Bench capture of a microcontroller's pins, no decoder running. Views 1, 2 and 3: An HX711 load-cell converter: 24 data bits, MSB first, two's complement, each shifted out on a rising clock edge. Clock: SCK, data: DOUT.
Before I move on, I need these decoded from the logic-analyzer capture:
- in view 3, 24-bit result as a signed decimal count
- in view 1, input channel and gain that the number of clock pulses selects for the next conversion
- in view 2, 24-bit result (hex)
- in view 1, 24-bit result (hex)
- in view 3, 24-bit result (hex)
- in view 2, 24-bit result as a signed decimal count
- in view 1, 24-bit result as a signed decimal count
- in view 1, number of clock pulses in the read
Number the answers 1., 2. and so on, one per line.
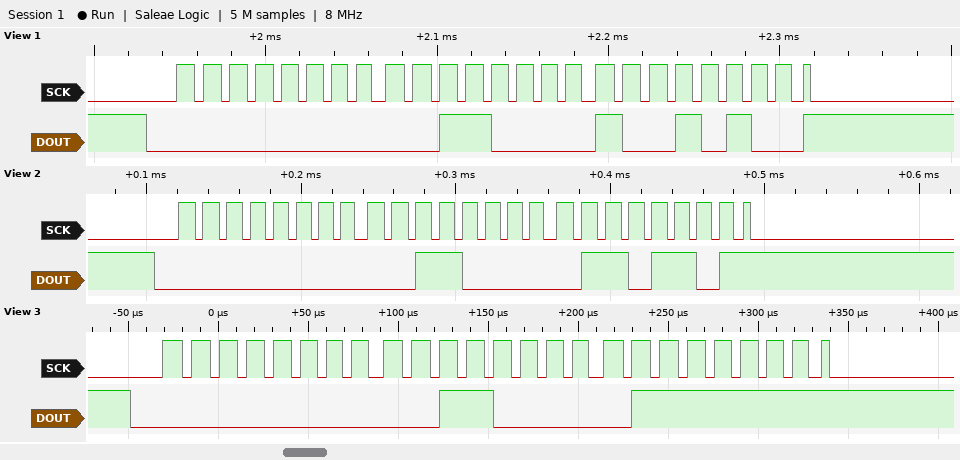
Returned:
1. 12415
2. channel A, gain 128
3. 0x00306D
4. 0x003094
5. 0x00307F
6. 12397
7. 12436
8. 25
